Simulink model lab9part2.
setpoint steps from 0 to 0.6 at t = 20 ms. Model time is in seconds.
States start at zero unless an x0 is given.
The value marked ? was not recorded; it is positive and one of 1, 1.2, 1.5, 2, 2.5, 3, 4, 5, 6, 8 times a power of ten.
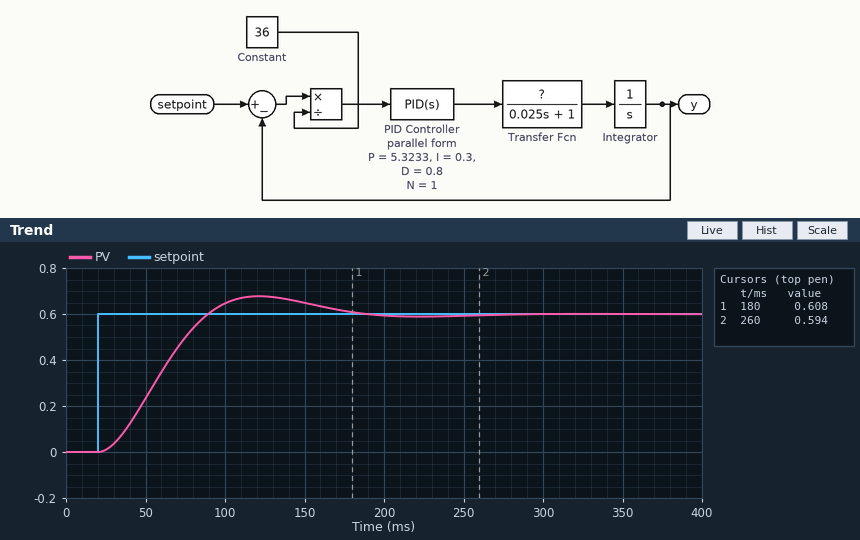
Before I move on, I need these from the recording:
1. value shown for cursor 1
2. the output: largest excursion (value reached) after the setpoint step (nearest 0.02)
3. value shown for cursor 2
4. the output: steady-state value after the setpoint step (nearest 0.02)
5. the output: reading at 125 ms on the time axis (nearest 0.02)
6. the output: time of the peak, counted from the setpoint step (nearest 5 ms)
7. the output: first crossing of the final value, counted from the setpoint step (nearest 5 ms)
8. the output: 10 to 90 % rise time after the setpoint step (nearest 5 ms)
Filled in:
0.608
0.68
0.594
0.60
0.68
100 ms
70 ms
45 ms
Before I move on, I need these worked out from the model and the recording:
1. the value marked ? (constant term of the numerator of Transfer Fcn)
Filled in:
200
